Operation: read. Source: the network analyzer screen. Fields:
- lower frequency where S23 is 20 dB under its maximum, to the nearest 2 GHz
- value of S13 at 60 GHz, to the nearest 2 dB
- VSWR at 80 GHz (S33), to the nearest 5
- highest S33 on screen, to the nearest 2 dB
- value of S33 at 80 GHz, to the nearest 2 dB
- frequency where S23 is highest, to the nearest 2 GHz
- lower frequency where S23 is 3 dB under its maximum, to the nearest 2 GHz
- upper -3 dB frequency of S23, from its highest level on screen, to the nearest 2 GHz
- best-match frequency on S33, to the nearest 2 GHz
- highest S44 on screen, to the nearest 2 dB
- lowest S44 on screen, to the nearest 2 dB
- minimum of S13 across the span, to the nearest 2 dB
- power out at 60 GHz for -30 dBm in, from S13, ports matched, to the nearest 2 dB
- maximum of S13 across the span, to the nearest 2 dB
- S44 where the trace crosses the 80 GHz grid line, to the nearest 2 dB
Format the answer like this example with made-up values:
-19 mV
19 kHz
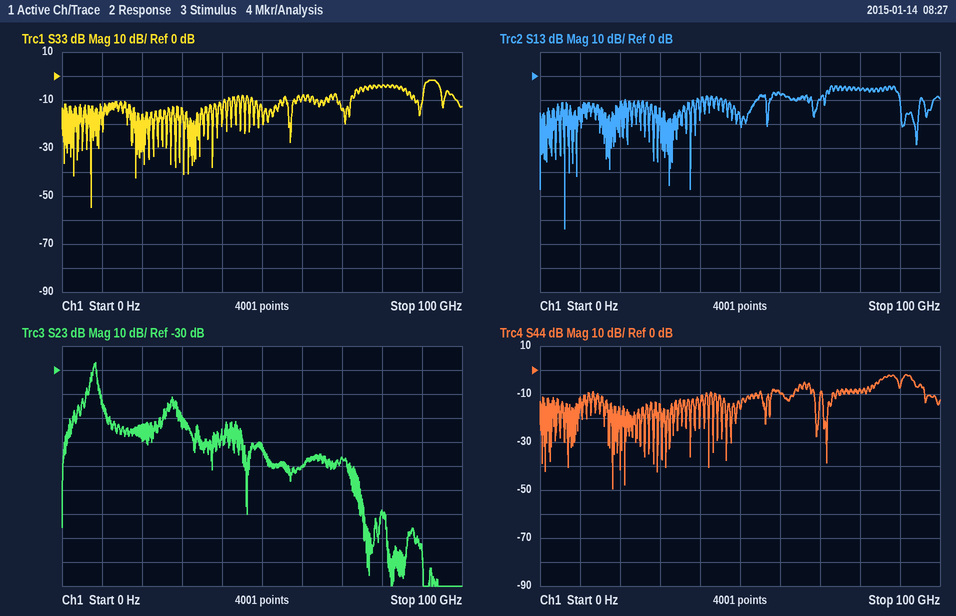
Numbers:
4 GHz
-8 dB
5
-2 dB
-4 dB
8 GHz
8 GHz
8 GHz
8 GHz
-2 dB
-50 dB
-64 dB
-38 dBm
-4 dB
-8 dB
